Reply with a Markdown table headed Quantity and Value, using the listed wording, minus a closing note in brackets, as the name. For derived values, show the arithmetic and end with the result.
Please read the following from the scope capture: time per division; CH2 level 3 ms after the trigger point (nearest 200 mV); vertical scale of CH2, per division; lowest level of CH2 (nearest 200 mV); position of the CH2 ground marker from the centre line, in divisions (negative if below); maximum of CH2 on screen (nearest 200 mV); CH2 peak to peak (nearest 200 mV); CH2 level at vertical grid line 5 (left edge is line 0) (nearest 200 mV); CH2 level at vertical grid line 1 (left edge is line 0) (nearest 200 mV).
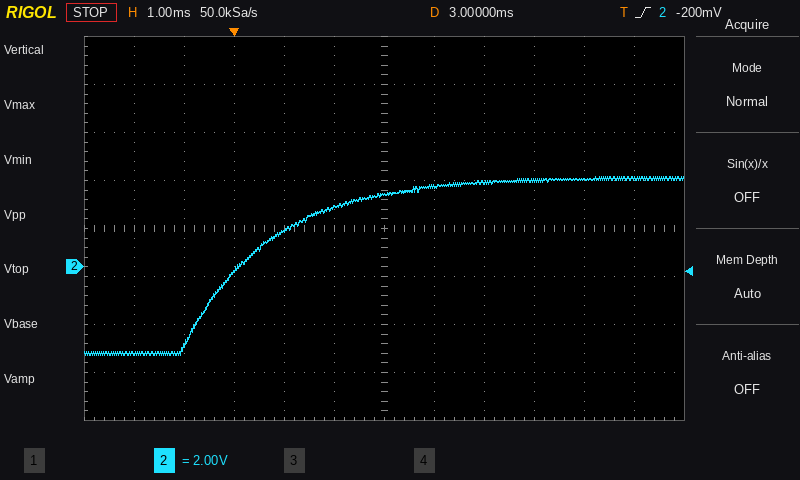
| Quantity | Value |
|---|---|
| time per division | 1 ms |
| CH2 level 3 ms after the trigger point | 3.0 V |
| vertical scale of CH2, per division | 2 V |
| lowest level of CH2 | -3.6 V |
| position of the CH2 ground marker from the centre line, in divisions | -0.8 div |
| maximum of CH2 on screen | 3.8 V |
| CH2 peak to peak | 3.8 V − (-3.6 V) = 7.4 V |
| CH2 level at vertical grid line 5 (left edge is line 0) | 2.4 V |
| CH2 level at vertical grid line 1 (left edge is line 0) | -3.6 V |
